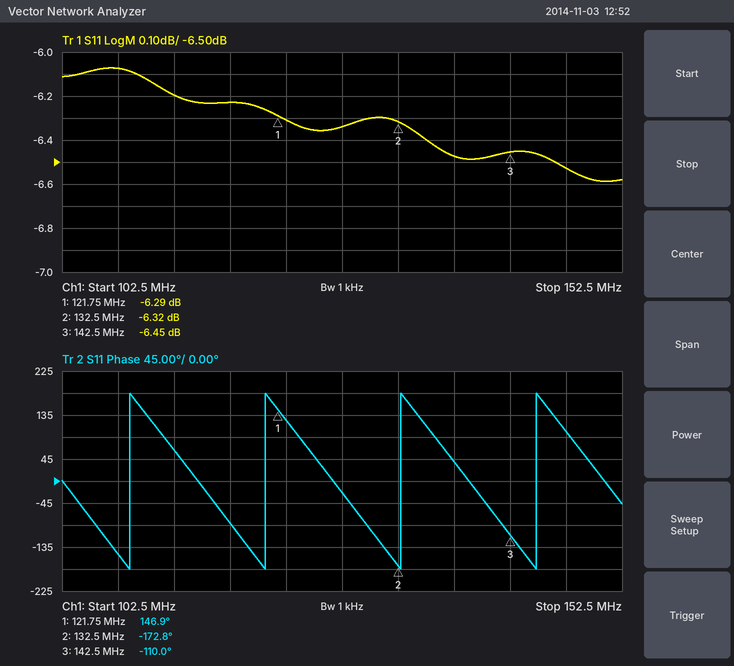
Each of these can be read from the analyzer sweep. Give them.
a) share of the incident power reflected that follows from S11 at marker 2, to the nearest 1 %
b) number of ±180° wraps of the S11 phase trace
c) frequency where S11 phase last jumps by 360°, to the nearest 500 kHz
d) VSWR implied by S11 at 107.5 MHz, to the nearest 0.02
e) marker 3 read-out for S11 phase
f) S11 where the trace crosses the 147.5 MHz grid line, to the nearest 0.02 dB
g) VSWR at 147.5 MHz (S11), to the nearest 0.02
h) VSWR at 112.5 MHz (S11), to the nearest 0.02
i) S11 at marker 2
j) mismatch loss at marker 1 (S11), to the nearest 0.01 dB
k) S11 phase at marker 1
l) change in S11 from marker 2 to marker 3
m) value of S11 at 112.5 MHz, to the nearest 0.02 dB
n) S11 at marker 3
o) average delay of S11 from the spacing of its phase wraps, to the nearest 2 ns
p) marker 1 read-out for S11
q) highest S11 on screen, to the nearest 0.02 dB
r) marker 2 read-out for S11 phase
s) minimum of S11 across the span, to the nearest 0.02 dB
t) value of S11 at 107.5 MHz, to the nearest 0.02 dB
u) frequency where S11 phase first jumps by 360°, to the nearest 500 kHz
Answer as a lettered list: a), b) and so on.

a) 23 %
b) 4
c) 145.0 MHz
d) 2.98
e) -110.0°
f) -6.52 dB
g) 2.78
h) 2.92
i) -6.32 dB
j) 1.16 dB
k) 146.9°
l) -0.13 dB
m) -6.20 dB
n) -6.45 dB
o) 82 ns
p) -6.29 dB
q) -6.08 dB
r) -172.8°
s) -6.58 dB
t) -6.08 dB
u) 108.5 MHz
